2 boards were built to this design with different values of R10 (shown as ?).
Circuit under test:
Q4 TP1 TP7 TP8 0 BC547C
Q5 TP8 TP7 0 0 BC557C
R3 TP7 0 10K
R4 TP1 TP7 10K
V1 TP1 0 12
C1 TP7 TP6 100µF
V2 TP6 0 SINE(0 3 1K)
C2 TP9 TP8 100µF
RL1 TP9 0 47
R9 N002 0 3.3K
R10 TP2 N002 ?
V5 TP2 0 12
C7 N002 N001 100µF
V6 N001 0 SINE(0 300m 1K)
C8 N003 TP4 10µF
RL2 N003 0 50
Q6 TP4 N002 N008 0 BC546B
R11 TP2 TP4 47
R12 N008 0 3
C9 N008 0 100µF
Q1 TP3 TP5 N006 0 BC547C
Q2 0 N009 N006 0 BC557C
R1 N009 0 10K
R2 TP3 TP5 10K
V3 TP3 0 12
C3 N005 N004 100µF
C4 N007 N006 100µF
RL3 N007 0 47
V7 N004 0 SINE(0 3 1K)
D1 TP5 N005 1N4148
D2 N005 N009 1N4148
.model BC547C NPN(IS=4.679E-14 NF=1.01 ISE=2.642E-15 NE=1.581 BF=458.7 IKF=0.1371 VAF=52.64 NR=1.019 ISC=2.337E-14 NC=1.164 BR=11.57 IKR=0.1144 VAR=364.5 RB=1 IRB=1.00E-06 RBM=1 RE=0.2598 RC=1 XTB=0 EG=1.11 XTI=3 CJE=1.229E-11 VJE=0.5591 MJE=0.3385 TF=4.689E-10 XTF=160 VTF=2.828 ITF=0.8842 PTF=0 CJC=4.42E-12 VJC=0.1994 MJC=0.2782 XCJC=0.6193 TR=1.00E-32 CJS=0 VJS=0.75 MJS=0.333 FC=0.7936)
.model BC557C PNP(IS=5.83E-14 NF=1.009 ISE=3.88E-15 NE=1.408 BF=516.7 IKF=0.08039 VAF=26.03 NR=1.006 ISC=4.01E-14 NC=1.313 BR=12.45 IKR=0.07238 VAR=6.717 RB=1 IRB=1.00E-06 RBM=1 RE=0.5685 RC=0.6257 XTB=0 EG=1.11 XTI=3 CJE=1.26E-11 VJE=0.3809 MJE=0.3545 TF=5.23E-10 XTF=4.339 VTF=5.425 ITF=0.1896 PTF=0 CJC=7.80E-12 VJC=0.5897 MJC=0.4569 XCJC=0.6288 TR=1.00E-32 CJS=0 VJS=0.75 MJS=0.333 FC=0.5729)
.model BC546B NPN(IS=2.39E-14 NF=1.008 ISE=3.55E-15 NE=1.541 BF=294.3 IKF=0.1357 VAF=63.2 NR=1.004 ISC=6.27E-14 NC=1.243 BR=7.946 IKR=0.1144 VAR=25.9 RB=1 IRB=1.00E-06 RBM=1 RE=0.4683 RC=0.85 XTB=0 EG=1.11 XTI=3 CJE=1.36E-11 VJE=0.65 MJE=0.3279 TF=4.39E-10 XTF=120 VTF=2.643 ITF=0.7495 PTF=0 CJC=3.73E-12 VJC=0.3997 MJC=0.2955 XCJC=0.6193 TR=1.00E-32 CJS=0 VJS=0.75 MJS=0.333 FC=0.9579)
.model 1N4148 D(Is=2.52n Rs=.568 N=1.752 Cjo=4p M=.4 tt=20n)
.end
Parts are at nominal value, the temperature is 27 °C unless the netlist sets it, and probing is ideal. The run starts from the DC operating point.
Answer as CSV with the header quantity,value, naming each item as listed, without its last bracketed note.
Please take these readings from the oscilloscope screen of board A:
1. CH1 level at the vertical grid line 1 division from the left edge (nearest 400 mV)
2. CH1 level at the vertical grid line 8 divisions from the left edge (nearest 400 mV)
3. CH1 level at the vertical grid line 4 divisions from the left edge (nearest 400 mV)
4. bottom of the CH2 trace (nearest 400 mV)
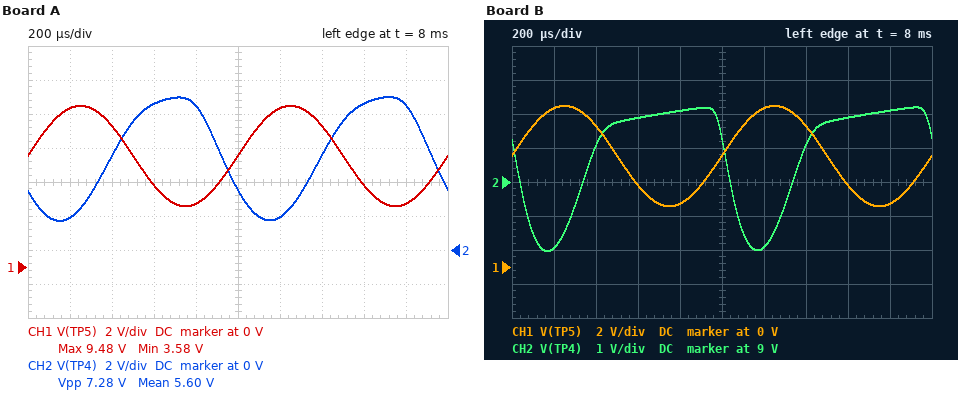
quantity,value
CH1 level at the vertical grid line 1 division from the left edge,9.2 V
CH1 level at the vertical grid line 8 divisions from the left edge,4.8 V
CH1 level at the vertical grid line 4 divisions from the left edge,3.6 V
bottom of the CH2 trace,1.6 V
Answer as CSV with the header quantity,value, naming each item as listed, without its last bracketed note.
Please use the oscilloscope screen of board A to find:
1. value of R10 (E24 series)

quantity,value
value of R10,8.2 kΩ
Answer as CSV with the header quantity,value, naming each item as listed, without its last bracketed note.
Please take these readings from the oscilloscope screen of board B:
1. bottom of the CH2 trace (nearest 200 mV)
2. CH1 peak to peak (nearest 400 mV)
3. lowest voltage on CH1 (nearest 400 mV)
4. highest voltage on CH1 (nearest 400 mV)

quantity,value
bottom of the CH2 trace,7.0 V
CH1 peak to peak,6.0 V
lowest voltage on CH1,3.6 V
highest voltage on CH1,9.6 V
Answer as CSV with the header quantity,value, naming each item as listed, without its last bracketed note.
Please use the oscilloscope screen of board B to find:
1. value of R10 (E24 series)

quantity,value
value of R10,33 kΩ
